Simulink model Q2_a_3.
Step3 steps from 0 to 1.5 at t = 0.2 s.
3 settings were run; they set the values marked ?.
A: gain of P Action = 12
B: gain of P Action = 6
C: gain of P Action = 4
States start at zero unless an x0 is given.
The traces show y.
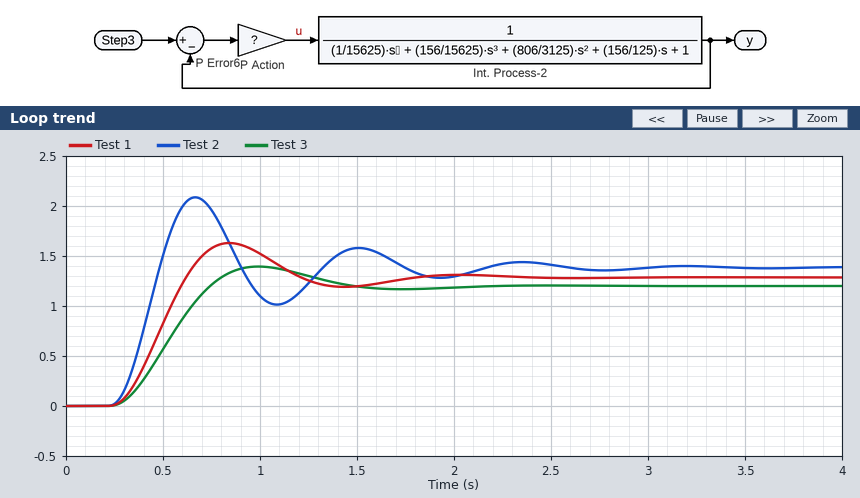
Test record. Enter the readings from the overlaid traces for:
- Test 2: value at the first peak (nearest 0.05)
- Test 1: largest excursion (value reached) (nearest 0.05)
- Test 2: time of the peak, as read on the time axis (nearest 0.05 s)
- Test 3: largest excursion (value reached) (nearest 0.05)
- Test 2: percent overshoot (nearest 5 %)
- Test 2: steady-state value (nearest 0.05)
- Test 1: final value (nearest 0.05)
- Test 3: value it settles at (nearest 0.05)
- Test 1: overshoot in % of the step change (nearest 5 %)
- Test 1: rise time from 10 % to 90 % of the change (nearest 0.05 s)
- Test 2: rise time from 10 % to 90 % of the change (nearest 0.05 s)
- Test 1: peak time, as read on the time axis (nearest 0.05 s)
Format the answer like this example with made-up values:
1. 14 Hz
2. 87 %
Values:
1. 2.10
2. 1.65
3. 0.65 s
4. 1.40
5. 50 %
6. 1.40
7. 1.30
8. 1.20
9. 25 %
10. 0.25 s
11. 0.15 s
12. 0.85 s
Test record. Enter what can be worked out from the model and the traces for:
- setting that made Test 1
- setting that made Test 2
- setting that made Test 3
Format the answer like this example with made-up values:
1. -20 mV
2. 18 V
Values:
1. B
2. A
3. C
